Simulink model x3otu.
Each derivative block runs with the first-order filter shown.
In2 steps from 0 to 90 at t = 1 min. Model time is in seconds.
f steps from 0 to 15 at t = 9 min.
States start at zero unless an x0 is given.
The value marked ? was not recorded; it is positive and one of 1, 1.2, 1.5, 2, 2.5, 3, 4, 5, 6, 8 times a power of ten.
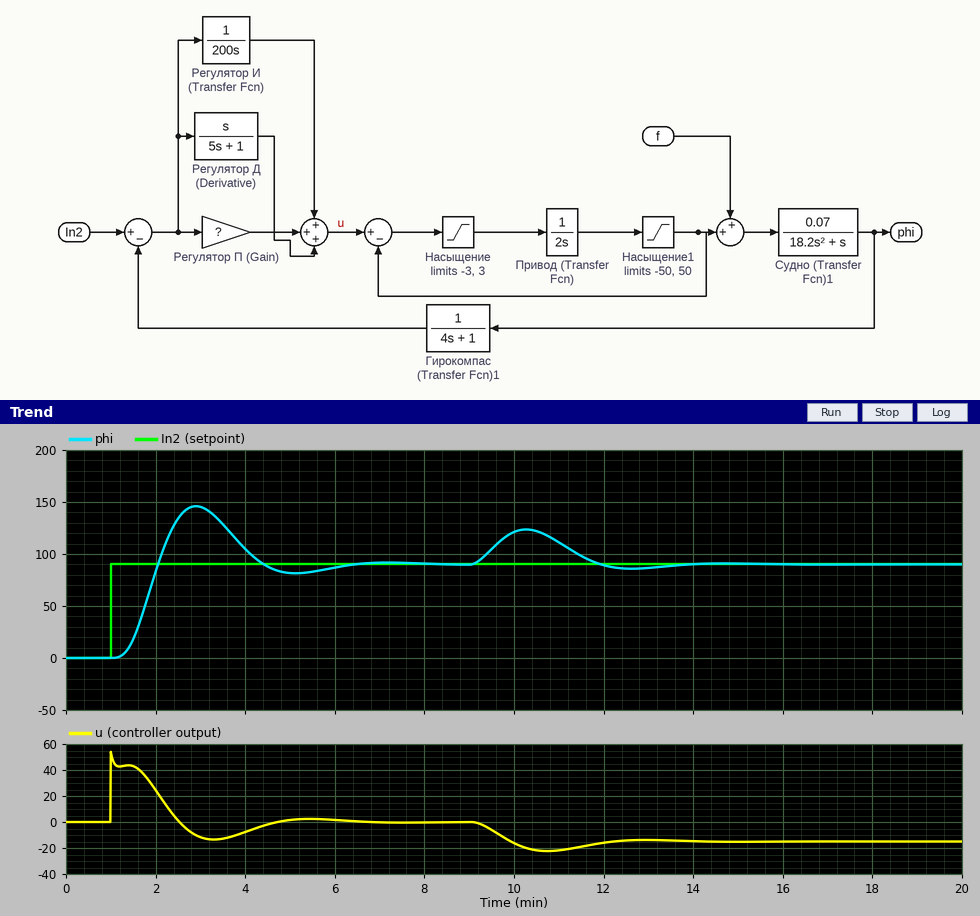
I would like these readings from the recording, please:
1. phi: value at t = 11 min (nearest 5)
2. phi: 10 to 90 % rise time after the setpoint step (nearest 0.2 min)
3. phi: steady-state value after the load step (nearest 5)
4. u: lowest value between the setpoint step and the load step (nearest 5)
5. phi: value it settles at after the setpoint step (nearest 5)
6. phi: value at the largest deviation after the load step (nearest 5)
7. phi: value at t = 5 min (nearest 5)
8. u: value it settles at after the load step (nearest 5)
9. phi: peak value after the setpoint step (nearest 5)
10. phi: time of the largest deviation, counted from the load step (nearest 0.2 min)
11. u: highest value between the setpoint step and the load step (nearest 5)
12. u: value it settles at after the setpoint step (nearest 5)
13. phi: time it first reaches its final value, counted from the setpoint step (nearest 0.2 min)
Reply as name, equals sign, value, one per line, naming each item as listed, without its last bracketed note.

phi: value at t = 11 min = 110
phi: 10 to 90 % rise time after the setpoint step = 0.6 min
phi: steady-state value after the load step = 90
u: lowest value between the setpoint step and the load step = -15
phi: value it settles at after the setpoint step = 90
phi: value at the largest deviation after the load step = 125
phi: value at t = 5 min = 80
u: value it settles at after the load step = -15
phi: peak value after the setpoint step = 145
phi: time of the largest deviation, counted from the load step = 1.2 min
u: highest value between the setpoint step and the load step = 55
u: value it settles at after the setpoint step = 0
phi: time it first reaches its final value, counted from the setpoint step = 1.0 min
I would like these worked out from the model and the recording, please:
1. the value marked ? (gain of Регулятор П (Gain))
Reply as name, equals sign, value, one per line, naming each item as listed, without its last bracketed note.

the value marked ? (gain of Регулятор П (Gain)) = 0.4
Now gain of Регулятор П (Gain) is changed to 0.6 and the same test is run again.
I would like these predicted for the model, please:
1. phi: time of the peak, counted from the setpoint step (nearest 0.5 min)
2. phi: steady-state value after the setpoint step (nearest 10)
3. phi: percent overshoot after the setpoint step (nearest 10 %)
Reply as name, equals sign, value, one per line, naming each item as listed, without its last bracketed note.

phi: time of the peak, counted from the setpoint step = 1.5 min
phi: steady-state value after the setpoint step = 90
phi: percent overshoot after the setpoint step = 70 %
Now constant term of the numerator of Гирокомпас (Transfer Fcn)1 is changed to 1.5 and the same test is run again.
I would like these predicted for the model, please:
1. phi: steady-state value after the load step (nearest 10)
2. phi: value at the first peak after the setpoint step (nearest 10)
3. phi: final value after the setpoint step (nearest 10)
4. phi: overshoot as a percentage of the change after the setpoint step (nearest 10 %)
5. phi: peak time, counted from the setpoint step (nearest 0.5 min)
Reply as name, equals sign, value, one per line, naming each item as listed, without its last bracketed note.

phi: steady-state value after the load step = 60
phi: value at the first peak after the setpoint step = 100
phi: final value after the setpoint step = 60
phi: overshoot as a percentage of the change after the setpoint step = 70 %
phi: peak time, counted from the setpoint step = 1.5 min
